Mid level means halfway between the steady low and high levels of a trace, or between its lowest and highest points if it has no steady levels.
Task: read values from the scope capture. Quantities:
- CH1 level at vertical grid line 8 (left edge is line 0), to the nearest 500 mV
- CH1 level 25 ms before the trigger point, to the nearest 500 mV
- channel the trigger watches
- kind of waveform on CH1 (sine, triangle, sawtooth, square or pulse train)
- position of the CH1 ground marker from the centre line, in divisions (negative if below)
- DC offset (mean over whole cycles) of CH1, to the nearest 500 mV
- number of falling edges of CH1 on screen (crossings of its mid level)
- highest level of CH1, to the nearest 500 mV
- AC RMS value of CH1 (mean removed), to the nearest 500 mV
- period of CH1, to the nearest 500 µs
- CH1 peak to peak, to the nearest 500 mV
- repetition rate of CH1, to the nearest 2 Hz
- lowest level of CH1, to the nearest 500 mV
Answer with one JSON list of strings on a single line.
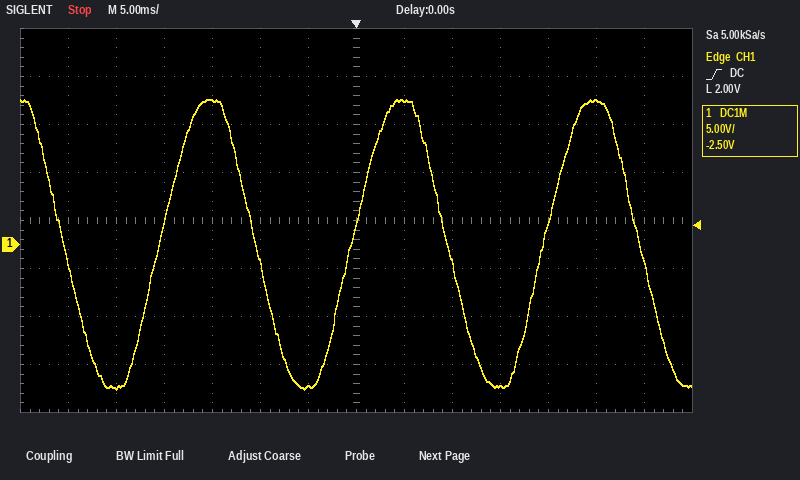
["15.0 V", "-15.0 V", "CH1", "sine", "-0.5 div", "0.0 V", "4", "15.0 V", "10.5 V", "20.0 ms", "30.0 V", "50 Hz", "-15.0 V"]
